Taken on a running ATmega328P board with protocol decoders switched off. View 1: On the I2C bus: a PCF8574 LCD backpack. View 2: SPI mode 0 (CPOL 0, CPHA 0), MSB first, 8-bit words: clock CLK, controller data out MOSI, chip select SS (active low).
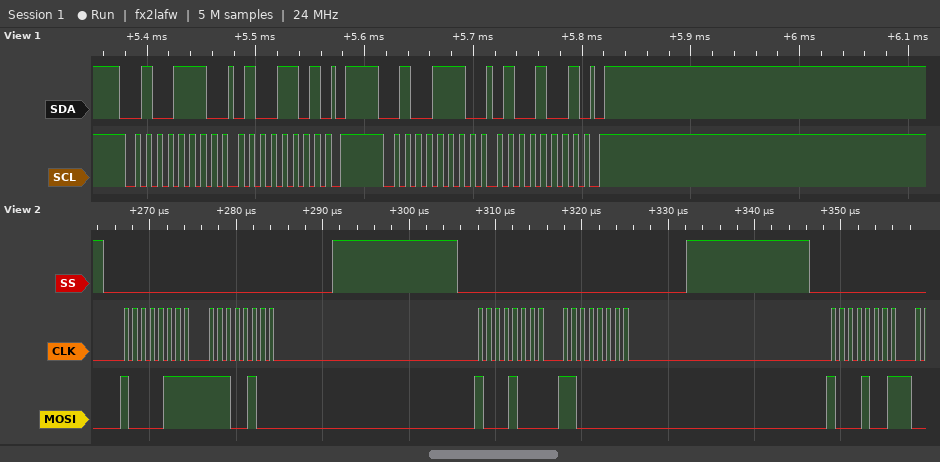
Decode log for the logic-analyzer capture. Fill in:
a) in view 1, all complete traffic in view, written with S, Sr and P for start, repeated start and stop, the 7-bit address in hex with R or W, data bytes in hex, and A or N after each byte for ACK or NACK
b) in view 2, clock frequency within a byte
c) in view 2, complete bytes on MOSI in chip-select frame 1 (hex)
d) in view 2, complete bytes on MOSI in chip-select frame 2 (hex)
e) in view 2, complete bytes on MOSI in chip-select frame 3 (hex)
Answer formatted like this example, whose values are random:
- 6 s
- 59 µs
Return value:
- S 27W A 4D A P S 27W A 49 A P
- 1 MHz
- 0x87 0xE4
- 0x88 0xC0
- 0x89
